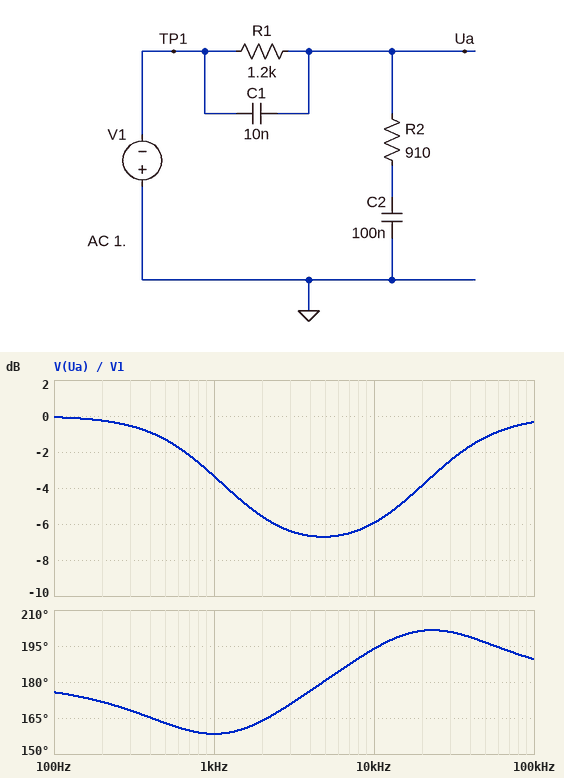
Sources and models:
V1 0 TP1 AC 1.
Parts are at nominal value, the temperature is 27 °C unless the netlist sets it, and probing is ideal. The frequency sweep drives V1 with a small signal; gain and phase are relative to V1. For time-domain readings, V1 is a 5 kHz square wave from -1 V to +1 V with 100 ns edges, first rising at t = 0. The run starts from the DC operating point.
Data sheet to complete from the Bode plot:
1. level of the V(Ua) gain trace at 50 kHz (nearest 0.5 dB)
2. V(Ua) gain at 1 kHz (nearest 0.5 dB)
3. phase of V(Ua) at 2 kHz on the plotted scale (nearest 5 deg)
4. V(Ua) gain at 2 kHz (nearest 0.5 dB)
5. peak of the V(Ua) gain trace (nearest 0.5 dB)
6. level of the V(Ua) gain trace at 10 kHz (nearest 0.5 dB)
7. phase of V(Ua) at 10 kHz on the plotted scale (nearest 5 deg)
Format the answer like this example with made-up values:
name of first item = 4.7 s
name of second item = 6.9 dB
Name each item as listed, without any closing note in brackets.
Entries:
level of the V(Ua) gain trace at 50 kHz = -1.0 dB
V(Ua) gain at 1 kHz = -3.5 dB
phase of V(Ua) at 2 kHz on the plotted scale = 165 deg
V(Ua) gain at 2 kHz = -5.5 dB
peak of the V(Ua) gain trace = 0 dB
level of the V(Ua) gain trace at 10 kHz = -6.0 dB
phase of V(Ua) at 10 kHz on the plotted scale = 195 deg
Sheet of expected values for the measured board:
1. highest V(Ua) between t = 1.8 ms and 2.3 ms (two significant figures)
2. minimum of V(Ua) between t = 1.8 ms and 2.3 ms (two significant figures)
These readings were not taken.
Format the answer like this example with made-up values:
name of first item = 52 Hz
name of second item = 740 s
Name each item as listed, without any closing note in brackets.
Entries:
highest V(Ua) between t = 1.8 ms and 2.3 ms = 1.4 V
minimum of V(Ua) between t = 1.8 ms and 2.3 ms = -1.4 V
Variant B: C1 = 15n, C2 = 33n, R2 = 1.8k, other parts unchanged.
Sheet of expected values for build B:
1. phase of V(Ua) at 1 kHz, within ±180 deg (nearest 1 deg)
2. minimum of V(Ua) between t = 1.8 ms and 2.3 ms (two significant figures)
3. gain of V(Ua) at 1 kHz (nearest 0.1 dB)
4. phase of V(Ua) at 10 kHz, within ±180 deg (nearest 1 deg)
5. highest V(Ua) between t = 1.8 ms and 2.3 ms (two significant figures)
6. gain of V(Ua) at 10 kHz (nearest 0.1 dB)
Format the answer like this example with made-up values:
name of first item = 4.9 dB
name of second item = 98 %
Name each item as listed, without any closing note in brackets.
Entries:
phase of V(Ua) at 1 kHz, within ±180 deg = 169 deg
minimum of V(Ua) between t = 1.8 ms and 2.3 ms = -1.2 V
gain of V(Ua) at 1 kHz = -1.0 dB
phase of V(Ua) at 10 kHz, within ±180 deg = -170 deg
highest V(Ua) between t = 1.8 ms and 2.3 ms = 1.2 V
gain of V(Ua) at 10 kHz = -2.8 dB
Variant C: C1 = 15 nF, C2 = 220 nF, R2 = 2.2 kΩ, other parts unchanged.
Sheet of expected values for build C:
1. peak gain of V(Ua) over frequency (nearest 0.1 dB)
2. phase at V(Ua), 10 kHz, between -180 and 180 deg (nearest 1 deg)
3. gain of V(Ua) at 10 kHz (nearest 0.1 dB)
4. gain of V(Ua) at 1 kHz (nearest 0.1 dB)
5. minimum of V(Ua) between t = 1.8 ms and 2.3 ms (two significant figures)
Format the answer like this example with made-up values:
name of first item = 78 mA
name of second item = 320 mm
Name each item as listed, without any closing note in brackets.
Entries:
peak gain of V(Ua) over frequency = 0 dB
phase at V(Ua), 10 kHz, between -180 and 180 deg = -168 deg
gain of V(Ua) at 10 kHz = -2.1 dB
gain of V(Ua) at 1 kHz = -3.6 dB
minimum of V(Ua) between t = 1.8 ms and 2.3 ms = -1.3 V
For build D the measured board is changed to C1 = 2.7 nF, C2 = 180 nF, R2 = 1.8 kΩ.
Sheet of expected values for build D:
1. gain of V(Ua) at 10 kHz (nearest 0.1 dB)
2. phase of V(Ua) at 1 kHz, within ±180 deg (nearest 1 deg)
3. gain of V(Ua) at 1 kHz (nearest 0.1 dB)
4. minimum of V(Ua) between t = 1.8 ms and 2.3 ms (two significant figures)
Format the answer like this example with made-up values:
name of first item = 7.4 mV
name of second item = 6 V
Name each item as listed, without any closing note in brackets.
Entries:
gain of V(Ua) at 10 kHz = -4.3 dB
phase of V(Ua) at 1 kHz, within ±180 deg = 171 deg
gain of V(Ua) at 1 kHz = -3.9 dB
minimum of V(Ua) between t = 1.8 ms and 2.3 ms = -1.3 V
